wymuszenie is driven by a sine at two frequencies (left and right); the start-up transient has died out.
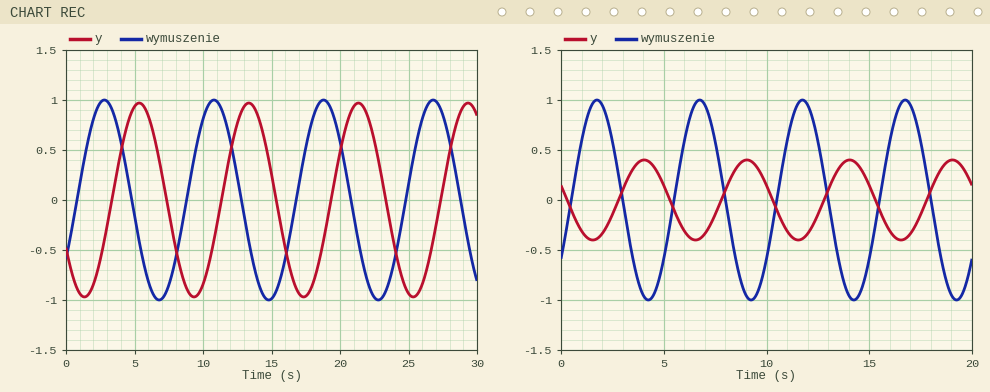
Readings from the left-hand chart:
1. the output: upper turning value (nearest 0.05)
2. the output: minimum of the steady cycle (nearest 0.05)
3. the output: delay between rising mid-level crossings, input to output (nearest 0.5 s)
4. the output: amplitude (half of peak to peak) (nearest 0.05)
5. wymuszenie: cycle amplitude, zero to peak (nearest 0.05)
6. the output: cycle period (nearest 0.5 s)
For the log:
0.95
-0.95
2.5 s
0.95
1.00
8.0 s
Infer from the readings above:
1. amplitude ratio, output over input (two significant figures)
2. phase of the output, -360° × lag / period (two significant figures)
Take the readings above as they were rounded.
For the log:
0.95
-110°
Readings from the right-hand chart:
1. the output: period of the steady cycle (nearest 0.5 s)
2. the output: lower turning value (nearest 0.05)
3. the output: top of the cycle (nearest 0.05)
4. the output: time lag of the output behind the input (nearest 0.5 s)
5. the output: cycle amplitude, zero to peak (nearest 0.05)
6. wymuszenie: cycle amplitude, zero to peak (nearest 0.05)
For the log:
5.0 s
-0.40
0.40
2.5 s
0.40
1.00
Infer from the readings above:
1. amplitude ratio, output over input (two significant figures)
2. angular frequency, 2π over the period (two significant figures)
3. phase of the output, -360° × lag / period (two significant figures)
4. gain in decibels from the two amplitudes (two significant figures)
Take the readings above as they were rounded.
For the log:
0.40
1.3 rad/s
-180°
-8.0 dB
